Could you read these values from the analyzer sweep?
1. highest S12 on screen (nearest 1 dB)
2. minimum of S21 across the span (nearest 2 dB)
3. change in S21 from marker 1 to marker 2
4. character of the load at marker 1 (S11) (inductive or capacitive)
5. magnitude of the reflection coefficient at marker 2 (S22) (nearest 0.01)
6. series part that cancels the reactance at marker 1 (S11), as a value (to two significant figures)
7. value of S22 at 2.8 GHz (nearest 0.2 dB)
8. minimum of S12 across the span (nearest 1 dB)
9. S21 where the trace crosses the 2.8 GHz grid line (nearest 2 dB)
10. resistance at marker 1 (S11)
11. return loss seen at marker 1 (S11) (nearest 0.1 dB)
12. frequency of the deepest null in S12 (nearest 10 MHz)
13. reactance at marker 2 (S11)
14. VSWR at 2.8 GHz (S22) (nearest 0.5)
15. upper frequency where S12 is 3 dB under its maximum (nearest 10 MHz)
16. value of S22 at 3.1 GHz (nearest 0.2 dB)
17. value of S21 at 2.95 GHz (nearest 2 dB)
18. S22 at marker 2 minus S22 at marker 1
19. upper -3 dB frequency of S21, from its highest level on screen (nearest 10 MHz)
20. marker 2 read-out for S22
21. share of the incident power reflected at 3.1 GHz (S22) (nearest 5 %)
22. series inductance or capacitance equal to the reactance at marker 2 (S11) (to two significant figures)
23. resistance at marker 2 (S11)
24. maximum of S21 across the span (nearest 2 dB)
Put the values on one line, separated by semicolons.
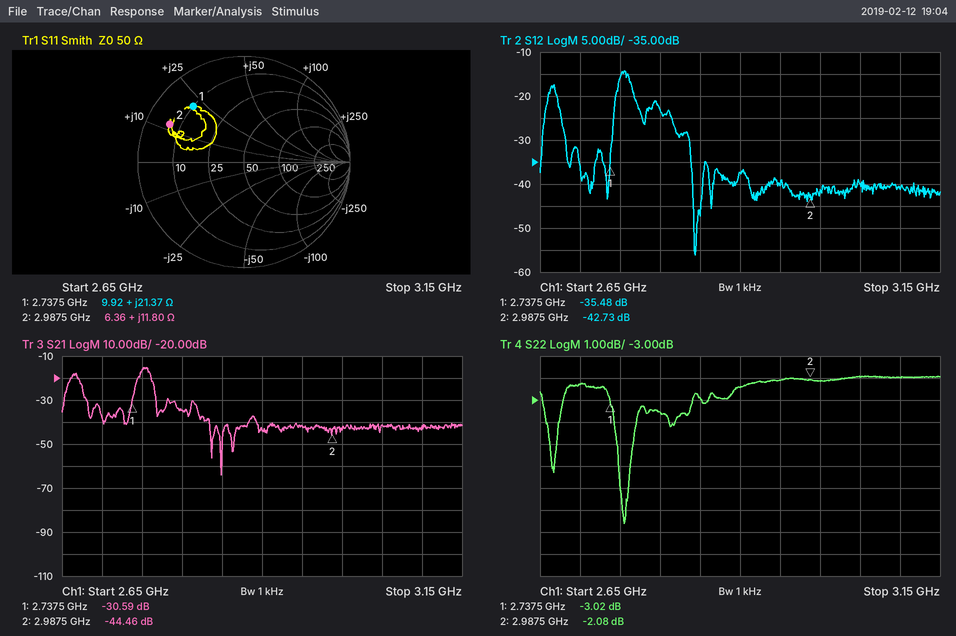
-14 dB; -64 dB; -13.87 dB; inductive; 0.79; 2.7 pF; -3.6 dB; -56 dB; -34 dB; 9.92 Ω; 2.9 dB; 2.84 GHz; +11.80 Ω; 5.0; 2.76 GHz; -2.0 dB; -42 dB; 0.94 dB; 2.76 GHz; -2.08 dB; 65 %; 630 pH; 6.36 Ω; -16 dB
